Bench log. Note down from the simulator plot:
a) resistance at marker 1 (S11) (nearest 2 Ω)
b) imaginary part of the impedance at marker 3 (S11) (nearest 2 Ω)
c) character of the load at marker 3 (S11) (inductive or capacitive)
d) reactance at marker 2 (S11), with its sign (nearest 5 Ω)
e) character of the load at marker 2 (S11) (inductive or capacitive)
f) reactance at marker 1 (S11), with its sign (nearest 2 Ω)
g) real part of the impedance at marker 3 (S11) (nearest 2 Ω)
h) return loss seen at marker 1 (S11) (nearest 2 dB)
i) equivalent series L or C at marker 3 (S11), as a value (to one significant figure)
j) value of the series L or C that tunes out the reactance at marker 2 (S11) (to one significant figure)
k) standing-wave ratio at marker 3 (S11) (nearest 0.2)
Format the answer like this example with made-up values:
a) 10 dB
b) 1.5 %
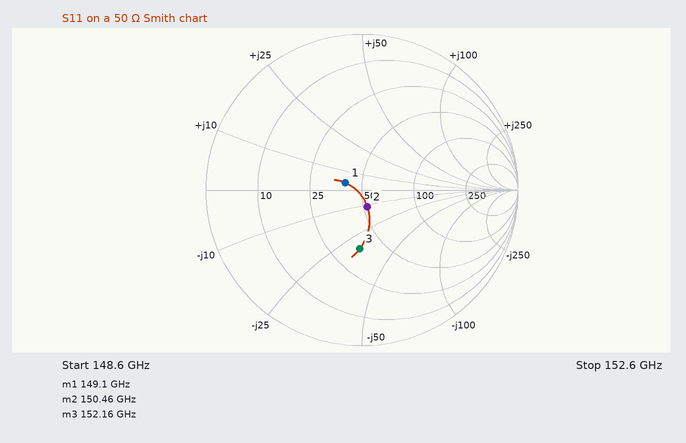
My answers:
a) 40 Ω
b) -32 Ω
c) capacitive
d) -10 Ω
e) capacitive
f) +4 Ω
g) 36 Ω
h) 18 dB
i) 30 fF
j) 10 pH
k) 2.2
